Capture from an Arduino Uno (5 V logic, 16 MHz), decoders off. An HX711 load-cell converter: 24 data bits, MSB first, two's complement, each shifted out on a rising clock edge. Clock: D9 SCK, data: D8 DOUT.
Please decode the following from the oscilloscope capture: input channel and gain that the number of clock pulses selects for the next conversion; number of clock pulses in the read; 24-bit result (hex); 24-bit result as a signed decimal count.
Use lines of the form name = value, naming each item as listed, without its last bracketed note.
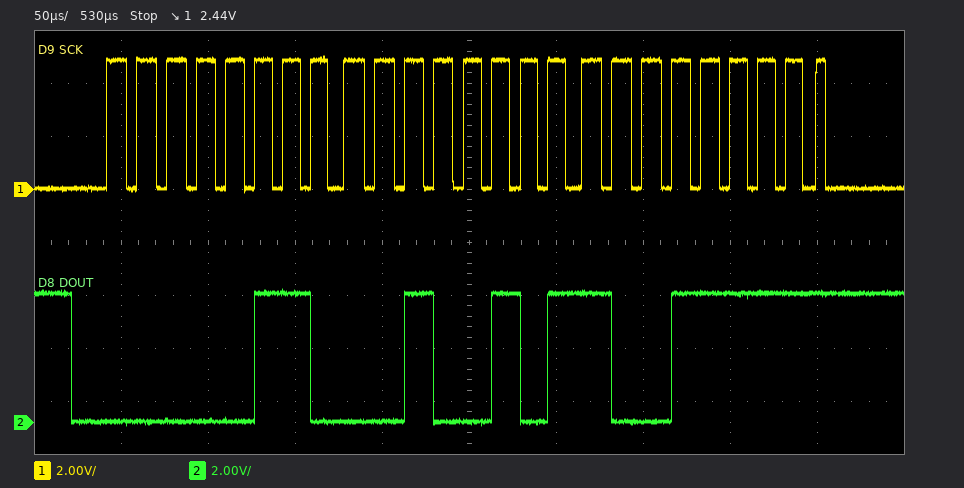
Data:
input channel and gain that the number of clock pulses selects for the next conversion = channel A, gain 128
number of clock pulses in the read = 25
24-bit result = 0x06259F
24-bit result as a signed decimal count = 402847
